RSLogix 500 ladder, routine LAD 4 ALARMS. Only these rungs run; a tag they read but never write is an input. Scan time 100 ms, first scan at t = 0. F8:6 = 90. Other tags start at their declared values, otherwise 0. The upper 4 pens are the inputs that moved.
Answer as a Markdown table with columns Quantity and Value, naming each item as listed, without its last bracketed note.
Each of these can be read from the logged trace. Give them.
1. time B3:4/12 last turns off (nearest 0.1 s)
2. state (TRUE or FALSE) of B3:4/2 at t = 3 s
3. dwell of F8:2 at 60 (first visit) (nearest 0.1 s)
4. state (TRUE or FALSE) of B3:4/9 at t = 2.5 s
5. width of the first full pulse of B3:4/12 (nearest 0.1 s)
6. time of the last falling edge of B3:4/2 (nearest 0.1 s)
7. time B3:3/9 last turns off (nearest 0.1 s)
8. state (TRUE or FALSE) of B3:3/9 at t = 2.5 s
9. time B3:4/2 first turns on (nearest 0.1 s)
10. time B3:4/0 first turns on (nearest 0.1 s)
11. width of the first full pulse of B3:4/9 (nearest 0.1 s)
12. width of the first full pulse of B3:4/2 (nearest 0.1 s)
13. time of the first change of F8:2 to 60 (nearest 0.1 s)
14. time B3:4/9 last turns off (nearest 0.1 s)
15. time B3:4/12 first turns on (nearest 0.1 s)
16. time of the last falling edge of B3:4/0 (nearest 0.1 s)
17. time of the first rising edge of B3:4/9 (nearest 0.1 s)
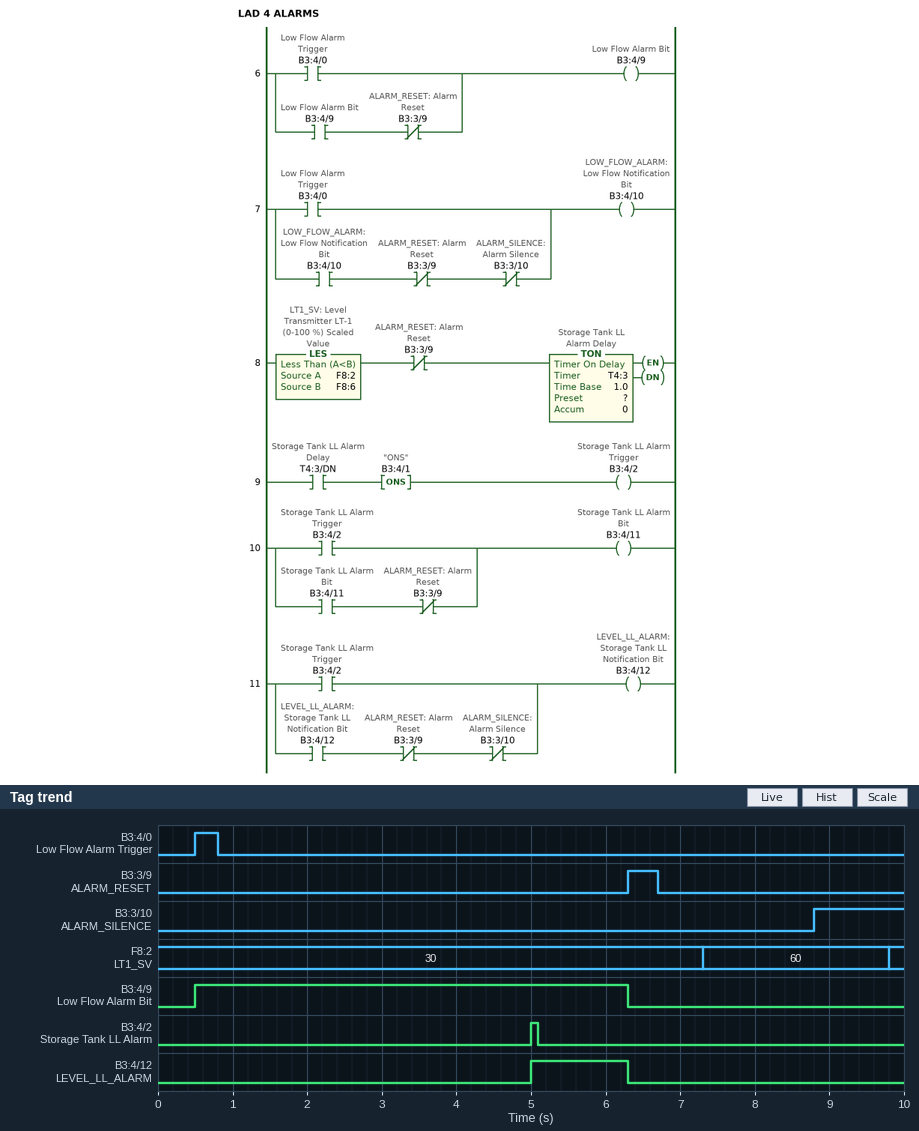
| Quantity | Value |
|---|---|
| time B3:4/12 last turns off | 6.3 s |
| state (TRUE or FALSE) of B3:4/2 at t = 3 s | FALSE |
| dwell of F8:2 at 60 (first visit) | 2.5 s |
| state (TRUE or FALSE) of B3:4/9 at t = 2.5 s | TRUE |
| width of the first full pulse of B3:4/12 | 1.3 s |
| time of the last falling edge of B3:4/2 | 5.1 s |
| time B3:3/9 last turns off | 6.7 s |
| state (TRUE or FALSE) of B3:3/9 at t = 2.5 s | FALSE |
| time B3:4/2 first turns on | 5.0 s |
| time B3:4/0 first turns on | 0.5 s |
| width of the first full pulse of B3:4/9 | 5.8 s |
| width of the first full pulse of B3:4/2 | 0.1 s |
| time of the first change of F8:2 to 60 | 7.3 s |
| time B3:4/9 last turns off | 6.3 s |
| time B3:4/12 first turns on | 5.0 s |
| time of the last falling edge of B3:4/0 | 0.8 s |
| time of the first rising edge of B3:4/9 | 0.5 s |
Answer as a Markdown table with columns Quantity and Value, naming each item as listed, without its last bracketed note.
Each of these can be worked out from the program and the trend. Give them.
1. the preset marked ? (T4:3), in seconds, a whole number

| Quantity | Value |
|---|---|
| the preset marked ? (T4:3), in seconds, a whole number | 5 s |
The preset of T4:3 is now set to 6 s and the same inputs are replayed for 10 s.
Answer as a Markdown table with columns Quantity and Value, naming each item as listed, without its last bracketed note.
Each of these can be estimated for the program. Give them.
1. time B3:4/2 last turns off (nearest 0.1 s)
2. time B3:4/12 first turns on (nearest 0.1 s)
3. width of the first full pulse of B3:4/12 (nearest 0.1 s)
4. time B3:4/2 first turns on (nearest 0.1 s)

| Quantity | Value |
|---|---|
| time B3:4/2 last turns off | 6.1 s |
| time B3:4/12 first turns on | 6.0 s |
| width of the first full pulse of B3:4/12 | 0.3 s |
| time B3:4/2 first turns on | 6.0 s |
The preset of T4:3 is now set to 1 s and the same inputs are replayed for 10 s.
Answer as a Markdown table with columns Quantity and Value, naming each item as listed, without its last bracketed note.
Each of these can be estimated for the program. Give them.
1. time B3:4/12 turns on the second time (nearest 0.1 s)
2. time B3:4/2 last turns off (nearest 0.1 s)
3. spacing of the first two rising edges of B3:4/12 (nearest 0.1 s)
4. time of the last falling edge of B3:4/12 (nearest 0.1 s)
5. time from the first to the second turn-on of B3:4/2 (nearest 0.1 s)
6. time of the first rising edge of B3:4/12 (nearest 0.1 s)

| Quantity | Value |
|---|---|
| time B3:4/12 turns on the second time | 7.7 s |
| time B3:4/2 last turns off | 7.8 s |
| spacing of the first two rising edges of B3:4/12 | 6.7 s |
| time of the last falling edge of B3:4/12 | 8.8 s |
| time from the first to the second turn-on of B3:4/2 | 6.7 s |
| time of the first rising edge of B3:4/12 | 1.0 s |
